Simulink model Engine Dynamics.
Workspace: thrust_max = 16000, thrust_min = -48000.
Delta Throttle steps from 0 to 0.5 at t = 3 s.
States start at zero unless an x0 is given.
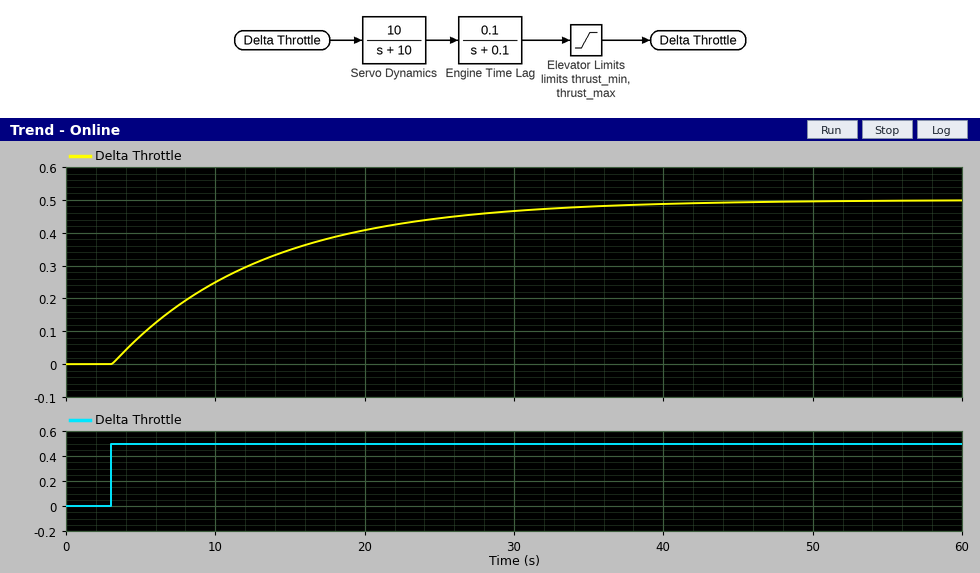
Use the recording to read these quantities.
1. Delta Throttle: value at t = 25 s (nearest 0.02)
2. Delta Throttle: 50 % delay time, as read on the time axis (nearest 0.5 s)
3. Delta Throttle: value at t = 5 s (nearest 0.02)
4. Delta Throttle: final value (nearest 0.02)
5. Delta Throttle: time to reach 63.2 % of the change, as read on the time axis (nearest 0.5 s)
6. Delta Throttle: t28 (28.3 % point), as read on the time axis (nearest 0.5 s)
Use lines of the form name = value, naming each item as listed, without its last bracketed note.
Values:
Delta Throttle: value at t = 25 s = 0.44
Delta Throttle: 50 % delay time, as read on the time axis = 10.0 s
Delta Throttle: value at t = 5 s = 0.08
Delta Throttle: final value = 0.50
Delta Throttle: time to reach 63.2 % of the change, as read on the time axis = 13.0 s
Delta Throttle: t28 (28.3 % point), as read on the time axis = 6.5 s
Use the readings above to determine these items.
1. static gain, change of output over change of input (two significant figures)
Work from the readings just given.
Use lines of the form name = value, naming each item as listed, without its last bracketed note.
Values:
static gain, change of output over change of input = 1.0
